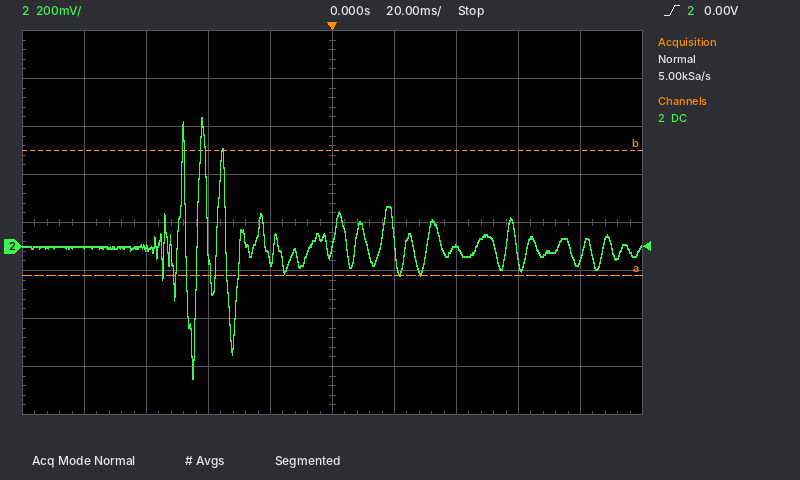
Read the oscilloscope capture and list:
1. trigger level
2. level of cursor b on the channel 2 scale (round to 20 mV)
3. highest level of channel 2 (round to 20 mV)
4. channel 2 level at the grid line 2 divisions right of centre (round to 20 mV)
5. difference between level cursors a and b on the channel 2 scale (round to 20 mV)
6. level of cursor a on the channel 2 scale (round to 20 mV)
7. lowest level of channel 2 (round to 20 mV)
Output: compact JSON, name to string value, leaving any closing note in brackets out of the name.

{"trigger level": "0.00 V", "level of cursor b on the channel 2 scale": "400 mV", "highest level of channel 2": "540 mV", "channel 2 level at the grid line 2 divisions right of centre": "0 mV", "difference between level cursors a and b on the channel 2 scale": "520 mV", "level of cursor a on the channel 2 scale": "-120 mV", "lowest level of channel 2": "-560 mV"}
